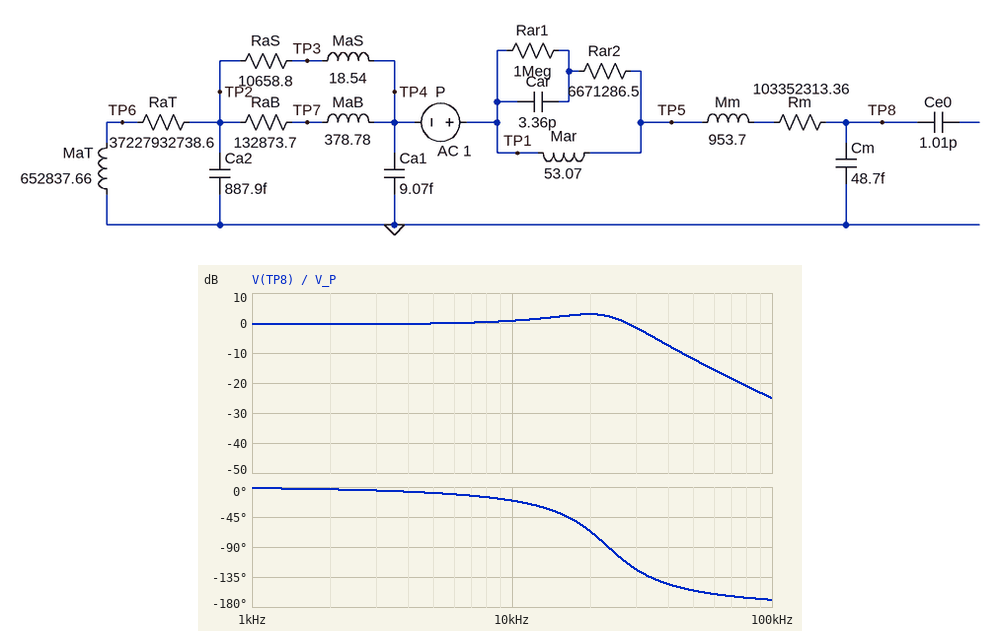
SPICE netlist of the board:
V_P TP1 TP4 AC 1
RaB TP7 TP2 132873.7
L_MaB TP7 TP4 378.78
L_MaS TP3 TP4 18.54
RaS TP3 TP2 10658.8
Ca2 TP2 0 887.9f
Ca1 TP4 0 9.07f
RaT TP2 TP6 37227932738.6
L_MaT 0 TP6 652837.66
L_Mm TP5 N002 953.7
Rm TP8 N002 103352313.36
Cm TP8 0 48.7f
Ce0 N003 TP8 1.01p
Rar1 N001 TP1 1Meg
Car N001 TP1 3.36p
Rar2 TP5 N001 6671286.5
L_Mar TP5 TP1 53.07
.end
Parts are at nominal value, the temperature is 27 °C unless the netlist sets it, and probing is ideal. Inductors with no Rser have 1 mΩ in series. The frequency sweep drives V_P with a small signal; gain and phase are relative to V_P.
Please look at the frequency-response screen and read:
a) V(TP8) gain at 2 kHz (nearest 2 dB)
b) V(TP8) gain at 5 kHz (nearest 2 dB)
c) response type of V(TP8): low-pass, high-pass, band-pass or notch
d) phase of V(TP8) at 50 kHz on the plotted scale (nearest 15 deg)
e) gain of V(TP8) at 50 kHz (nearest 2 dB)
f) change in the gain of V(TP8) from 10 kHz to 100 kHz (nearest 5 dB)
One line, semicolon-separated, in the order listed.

0 dB; 0 dB; low-pass; -150 deg; -12 dB; -25 dB
